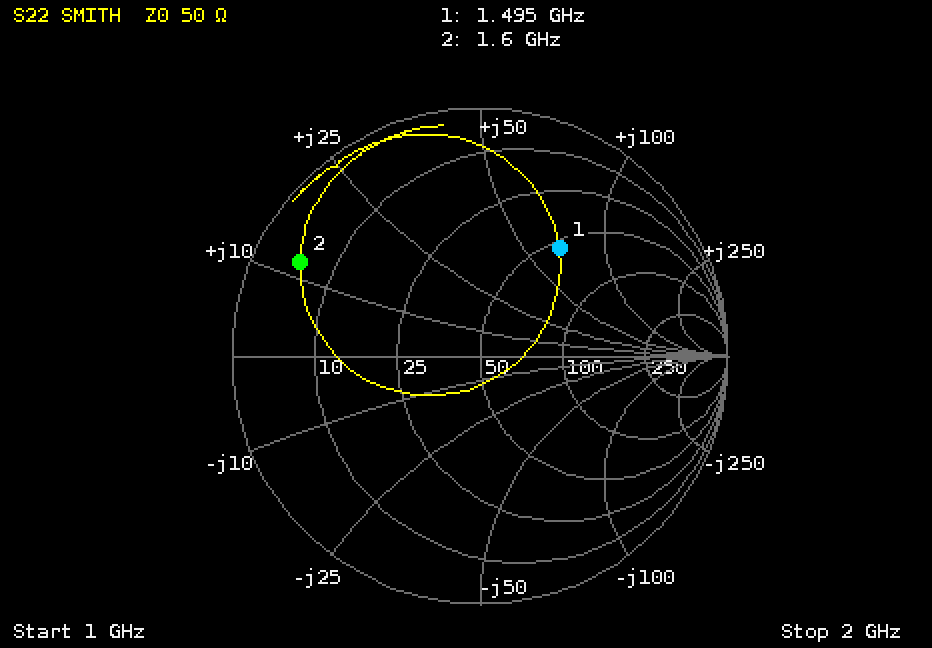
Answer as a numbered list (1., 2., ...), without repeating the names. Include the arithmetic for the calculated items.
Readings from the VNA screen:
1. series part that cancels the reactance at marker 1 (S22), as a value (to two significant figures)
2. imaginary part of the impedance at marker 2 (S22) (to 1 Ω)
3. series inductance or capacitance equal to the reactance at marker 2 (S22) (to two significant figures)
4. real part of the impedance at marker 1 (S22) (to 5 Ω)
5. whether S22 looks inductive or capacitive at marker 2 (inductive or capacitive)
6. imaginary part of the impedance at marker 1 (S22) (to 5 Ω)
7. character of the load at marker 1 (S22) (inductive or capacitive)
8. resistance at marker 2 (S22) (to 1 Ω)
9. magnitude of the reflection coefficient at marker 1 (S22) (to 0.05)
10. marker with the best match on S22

1. C = 1/(2π × 1.495 GHz × 65 Ω) ≈ 1.6 pF
2. +12 Ω
3. L = 12 Ω/(2π × 1.6 GHz) ≈ 1.2 nH
4. 55 Ω
5. inductive
6. +65 Ω
7. inductive
8. 5 Ω
9. 0.55
10. marker 1
